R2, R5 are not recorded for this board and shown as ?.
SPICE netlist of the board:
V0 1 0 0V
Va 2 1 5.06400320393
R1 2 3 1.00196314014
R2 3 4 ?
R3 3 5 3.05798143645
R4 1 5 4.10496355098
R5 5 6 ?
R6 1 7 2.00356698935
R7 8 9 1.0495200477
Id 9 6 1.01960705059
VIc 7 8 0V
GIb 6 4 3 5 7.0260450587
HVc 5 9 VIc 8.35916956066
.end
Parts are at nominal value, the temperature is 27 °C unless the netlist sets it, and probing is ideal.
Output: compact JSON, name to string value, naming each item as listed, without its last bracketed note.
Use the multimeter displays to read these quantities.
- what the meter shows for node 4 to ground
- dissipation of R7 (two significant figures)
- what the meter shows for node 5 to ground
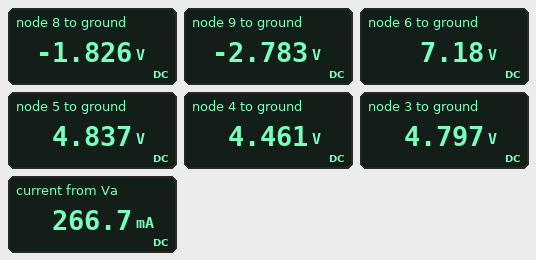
{"what the meter shows for node 4 to ground": "4.461 V", "dissipation of R7": "870 mW", "what the meter shows for node 5 to ground": "4.837 V"}
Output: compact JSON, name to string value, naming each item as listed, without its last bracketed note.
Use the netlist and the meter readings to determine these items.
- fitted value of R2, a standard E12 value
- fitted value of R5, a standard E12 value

{"fitted value of R2, a standard E12 value": "1.2 Ω", "fitted value of R5, a standard E12 value": "1.8 Ω"}
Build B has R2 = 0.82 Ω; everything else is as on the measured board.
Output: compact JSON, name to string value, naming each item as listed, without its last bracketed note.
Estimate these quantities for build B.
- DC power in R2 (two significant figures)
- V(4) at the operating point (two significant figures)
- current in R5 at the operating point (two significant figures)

{"DC power in R2": "64 mW", "V(4) at the operating point": "4.6 V", "current in R5 at the operating point": "1.3 A"}
